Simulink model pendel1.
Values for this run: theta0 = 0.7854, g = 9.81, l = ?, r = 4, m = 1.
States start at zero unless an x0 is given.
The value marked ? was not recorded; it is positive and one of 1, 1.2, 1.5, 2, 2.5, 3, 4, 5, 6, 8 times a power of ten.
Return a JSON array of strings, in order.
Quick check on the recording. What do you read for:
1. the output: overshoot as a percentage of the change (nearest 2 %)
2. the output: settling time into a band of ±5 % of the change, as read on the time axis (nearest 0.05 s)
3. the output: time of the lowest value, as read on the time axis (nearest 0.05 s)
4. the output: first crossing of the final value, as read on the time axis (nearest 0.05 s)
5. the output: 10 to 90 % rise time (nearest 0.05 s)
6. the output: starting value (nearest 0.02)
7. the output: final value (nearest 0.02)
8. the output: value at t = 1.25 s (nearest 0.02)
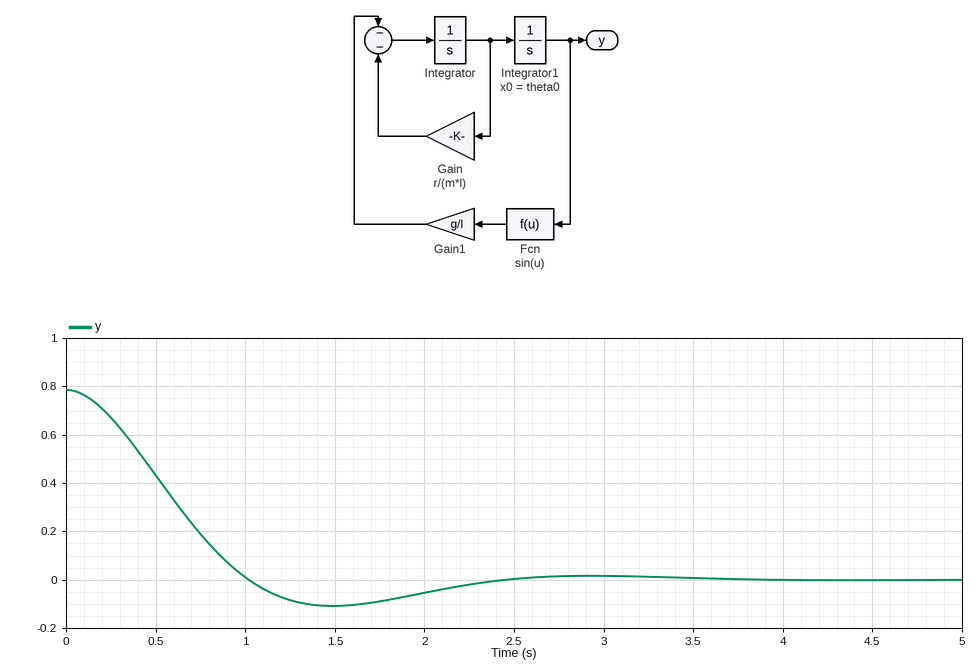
["14 %", "2.10 s", "1.50 s", "1.00 s", "0.70 s", "0.78", "0.00", "-0.08"]
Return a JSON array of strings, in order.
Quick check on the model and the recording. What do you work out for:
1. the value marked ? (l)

["1.5"]
